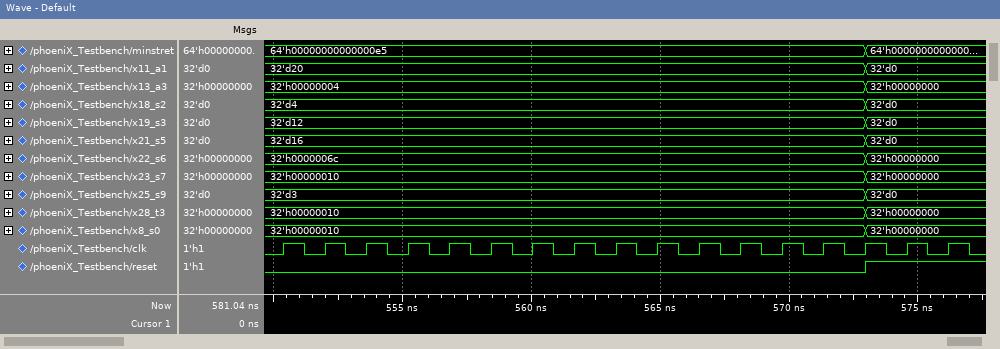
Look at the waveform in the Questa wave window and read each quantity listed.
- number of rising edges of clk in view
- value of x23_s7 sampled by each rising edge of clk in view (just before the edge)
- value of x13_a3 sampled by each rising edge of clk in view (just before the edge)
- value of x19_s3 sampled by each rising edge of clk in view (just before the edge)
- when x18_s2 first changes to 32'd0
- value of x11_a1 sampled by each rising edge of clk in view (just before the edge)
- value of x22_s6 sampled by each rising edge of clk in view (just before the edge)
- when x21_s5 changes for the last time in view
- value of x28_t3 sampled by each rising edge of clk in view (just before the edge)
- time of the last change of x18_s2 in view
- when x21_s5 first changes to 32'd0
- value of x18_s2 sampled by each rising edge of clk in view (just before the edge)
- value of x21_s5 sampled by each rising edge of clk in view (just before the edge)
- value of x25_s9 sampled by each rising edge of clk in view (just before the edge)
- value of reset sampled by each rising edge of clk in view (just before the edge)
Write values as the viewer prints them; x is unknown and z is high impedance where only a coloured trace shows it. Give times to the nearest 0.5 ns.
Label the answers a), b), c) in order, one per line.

a) 17
b) 32'h00000010, 32'h00000010, 32'h00000010, 32'h00000010, 32'h00000010, 32'h00000010, 32'h00000010, 32'h00000010, 32'h00000010, 32'h00000010, 32'h00000010, 32'h00000010, 32'h00000010, 32'h00000010, 32'h00000010, 32'h00000000, 32'h00000000
c) 32'h00000004, 32'h00000004, 32'h00000004, 32'h00000004, 32'h00000004, 32'h00000004, 32'h00000004, 32'h00000004, 32'h00000004, 32'h00000004, 32'h00000004, 32'h00000004, 32'h00000004, 32'h00000004, 32'h00000004, 32'h00000000, 32'h00000000
d) 32'd12, 32'd12, 32'd12, 32'd12, 32'd12, 32'd12, 32'd12, 32'd12, 32'd12, 32'd12, 32'd12, 32'd12, 32'd12, 32'd12, 32'd12, 32'd0, 32'd0
e) 573 ns
f) 32'd20, 32'd20, 32'd20, 32'd20, 32'd20, 32'd20, 32'd20, 32'd20, 32'd20, 32'd20, 32'd20, 32'd20, 32'd20, 32'd20, 32'd20, 32'd0, 32'd0
g) 32'h0000006c, 32'h0000006c, 32'h0000006c, 32'h0000006c, 32'h0000006c, 32'h0000006c, 32'h0000006c, 32'h0000006c, 32'h0000006c, 32'h0000006c, 32'h0000006c, 32'h0000006c, 32'h0000006c, 32'h0000006c, 32'h0000006c, 32'h00000000, 32'h00000000
h) 573 ns
i) 32'h00000010, 32'h00000010, 32'h00000010, 32'h00000010, 32'h00000010, 32'h00000010, 32'h00000010, 32'h00000010, 32'h00000010, 32'h00000010, 32'h00000010, 32'h00000010, 32'h00000010, 32'h00000010, 32'h00000010, 32'h00000000, 32'h00000000
j) 573 ns
k) 573 ns
l) 32'd4, 32'd4, 32'd4, 32'd4, 32'd4, 32'd4, 32'd4, 32'd4, 32'd4, 32'd4, 32'd4, 32'd4, 32'd4, 32'd4, 32'd4, 32'd0, 32'd0
m) 32'd16, 32'd16, 32'd16, 32'd16, 32'd16, 32'd16, 32'd16, 32'd16, 32'd16, 32'd16, 32'd16, 32'd16, 32'd16, 32'd16, 32'd16, 32'd0, 32'd0
n) 32'd3, 32'd3, 32'd3, 32'd3, 32'd3, 32'd3, 32'd3, 32'd3, 32'd3, 32'd3, 32'd3, 32'd3, 32'd3, 32'd3, 32'd3, 32'd0, 32'd0
o) 0 0 0 0 0 0 0 0 0 0 0 0 0 0 0 1 1
